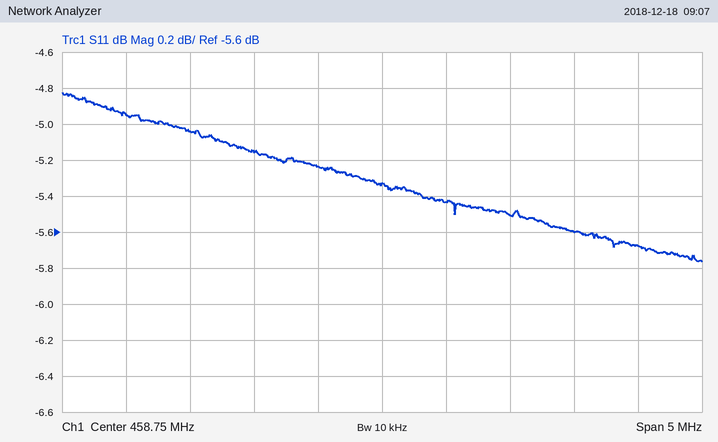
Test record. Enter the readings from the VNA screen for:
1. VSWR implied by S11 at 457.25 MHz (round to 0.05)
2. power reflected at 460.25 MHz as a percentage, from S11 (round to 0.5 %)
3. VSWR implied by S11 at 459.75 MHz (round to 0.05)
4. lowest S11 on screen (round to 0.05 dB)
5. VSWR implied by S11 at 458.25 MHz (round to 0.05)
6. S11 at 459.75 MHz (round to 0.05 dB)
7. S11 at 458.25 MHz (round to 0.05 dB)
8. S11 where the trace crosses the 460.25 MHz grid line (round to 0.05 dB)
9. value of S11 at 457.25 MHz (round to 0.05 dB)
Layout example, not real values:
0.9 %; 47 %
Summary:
3.55; 27.5 %; 3.25; -5.75 dB; 3.40; -5.50 dB; -5.25 dB; -5.60 dB; -5.05 dB
